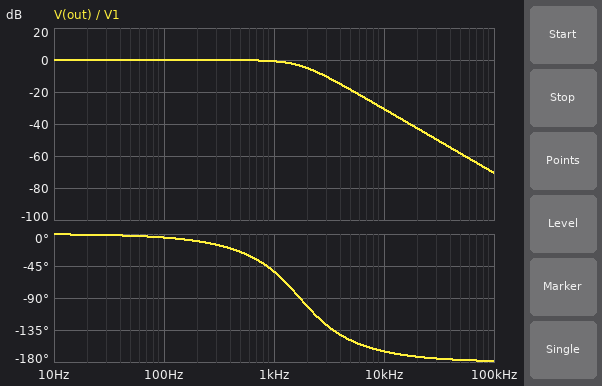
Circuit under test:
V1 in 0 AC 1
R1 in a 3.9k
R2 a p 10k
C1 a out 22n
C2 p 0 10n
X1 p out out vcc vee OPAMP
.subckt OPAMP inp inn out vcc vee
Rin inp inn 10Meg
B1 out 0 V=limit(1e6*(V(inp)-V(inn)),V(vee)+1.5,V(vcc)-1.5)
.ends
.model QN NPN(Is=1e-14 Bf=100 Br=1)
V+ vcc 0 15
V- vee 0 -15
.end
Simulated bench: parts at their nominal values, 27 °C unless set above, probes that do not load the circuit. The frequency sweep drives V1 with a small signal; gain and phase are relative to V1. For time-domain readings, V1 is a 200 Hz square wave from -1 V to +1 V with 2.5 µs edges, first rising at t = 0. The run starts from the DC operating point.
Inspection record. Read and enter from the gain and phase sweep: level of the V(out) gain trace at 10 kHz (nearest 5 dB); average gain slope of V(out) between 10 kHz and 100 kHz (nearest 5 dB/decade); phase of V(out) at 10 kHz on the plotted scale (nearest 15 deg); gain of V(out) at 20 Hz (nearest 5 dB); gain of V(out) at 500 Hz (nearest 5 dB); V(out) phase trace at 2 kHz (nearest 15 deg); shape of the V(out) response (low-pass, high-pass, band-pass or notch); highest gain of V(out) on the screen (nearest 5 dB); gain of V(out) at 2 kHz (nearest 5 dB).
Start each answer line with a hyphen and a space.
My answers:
- -30 dB
- -40 dB/decade
- -165 deg
- 0 dB
- 0 dB
- -105 deg
- low-pass
- 0 dB
- -5 dB
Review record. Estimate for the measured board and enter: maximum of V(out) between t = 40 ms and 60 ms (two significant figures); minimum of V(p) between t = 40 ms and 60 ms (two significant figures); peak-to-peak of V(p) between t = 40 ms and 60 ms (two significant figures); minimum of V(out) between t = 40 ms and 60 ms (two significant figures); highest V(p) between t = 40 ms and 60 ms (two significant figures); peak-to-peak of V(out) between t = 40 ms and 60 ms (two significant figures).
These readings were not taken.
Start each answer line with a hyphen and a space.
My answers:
- 1.1 V
- -1.1 V
- 2.1 V
- -1.1 V
- 1.1 V
- 2.1 V
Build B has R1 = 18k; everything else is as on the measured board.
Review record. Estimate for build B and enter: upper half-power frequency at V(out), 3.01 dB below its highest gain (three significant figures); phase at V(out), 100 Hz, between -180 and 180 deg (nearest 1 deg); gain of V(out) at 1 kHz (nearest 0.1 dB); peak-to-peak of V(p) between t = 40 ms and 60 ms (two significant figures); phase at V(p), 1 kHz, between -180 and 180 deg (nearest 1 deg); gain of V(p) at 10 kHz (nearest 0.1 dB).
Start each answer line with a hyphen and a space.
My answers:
- 804 Hz
- -10 deg
- -5.3 dB
- 2.2 V
- -108 deg
- -43.9 dB
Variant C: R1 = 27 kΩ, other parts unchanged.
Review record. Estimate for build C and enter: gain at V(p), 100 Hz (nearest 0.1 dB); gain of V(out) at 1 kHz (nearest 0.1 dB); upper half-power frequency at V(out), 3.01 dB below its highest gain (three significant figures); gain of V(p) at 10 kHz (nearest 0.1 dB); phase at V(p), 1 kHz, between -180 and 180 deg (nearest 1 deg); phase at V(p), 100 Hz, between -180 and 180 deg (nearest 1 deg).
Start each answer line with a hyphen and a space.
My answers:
- 0 dB
- -8.6 dB
- 605 Hz
- -47.4 dB
- -120 deg
- -13 deg
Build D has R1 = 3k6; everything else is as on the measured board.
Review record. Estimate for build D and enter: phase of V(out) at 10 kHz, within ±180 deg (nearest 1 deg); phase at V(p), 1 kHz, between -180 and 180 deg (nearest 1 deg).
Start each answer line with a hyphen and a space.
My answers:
- -164 deg
- -51 deg
